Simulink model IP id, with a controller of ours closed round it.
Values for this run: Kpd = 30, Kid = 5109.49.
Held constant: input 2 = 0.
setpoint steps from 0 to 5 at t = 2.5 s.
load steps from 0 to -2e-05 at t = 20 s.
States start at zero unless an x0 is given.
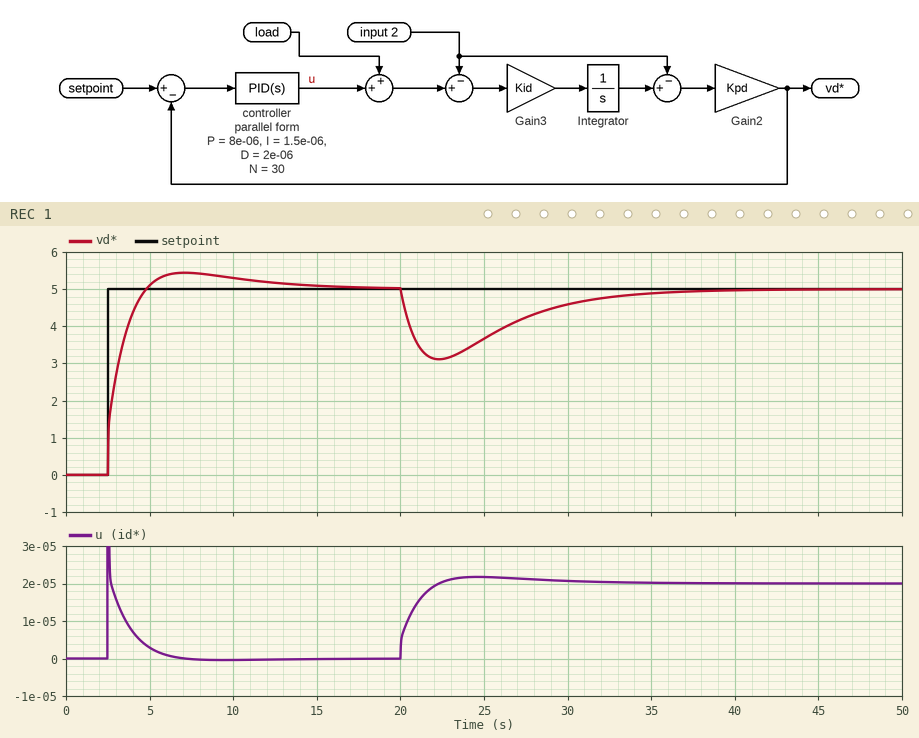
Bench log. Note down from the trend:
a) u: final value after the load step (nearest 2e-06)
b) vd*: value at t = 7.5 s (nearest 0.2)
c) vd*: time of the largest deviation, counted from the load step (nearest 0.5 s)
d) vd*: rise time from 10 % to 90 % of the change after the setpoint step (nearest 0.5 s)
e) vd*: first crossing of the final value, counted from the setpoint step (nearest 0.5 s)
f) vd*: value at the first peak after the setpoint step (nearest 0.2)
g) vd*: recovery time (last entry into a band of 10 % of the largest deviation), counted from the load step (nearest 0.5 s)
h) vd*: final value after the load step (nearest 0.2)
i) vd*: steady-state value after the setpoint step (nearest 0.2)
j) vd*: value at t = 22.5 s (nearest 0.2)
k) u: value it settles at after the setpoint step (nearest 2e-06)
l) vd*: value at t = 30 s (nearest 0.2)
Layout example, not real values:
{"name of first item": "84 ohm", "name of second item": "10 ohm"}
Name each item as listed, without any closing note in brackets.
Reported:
{"u: final value after the load step": "0.000020", "vd*: value at t = 7.5 s": "5.4", "vd*: time of the largest deviation, counted from the load step": "2.5 s", "vd*: rise time from 10 % to 90 % of the change after the setpoint step": "1.5 s", "vd*: first crossing of the final value, counted from the setpoint step": "2.5 s", "vd*: value at the first peak after the setpoint step": "5.4", "vd*: recovery time (last entry into a band of 10 % of the largest deviation), counted from the load step": "13.0 s", "vd*: final value after the load step": "5.0", "vd*: steady-state value after the setpoint step": "5.0", "vd*: value at t = 22.5 s": "3.2", "u: value it settles at after the setpoint step": "0.000000", "vd*: value at t = 30 s": "4.6"}
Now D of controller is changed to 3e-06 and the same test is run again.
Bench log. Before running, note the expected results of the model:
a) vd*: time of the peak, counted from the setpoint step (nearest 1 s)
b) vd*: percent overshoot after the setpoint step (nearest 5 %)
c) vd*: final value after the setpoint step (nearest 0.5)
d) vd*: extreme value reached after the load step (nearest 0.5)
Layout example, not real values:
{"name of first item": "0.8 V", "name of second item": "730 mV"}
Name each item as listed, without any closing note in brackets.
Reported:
{"vd*: time of the peak, counted from the setpoint step": "5 s", "vd*: percent overshoot after the setpoint step": "10 %", "vd*: final value after the setpoint step": "5.0", "vd*: extreme value reached after the load step": "3.0"}
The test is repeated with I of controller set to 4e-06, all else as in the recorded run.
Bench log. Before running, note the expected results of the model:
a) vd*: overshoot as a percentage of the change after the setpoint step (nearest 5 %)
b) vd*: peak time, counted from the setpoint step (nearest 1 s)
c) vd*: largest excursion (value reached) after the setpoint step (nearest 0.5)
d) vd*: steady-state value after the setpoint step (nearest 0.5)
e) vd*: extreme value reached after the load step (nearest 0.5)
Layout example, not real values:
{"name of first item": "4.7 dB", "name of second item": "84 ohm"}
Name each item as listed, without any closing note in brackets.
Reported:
{"vd*: overshoot as a percentage of the change after the setpoint step": "15 %", "vd*: peak time, counted from the setpoint step": "3 s", "vd*: largest excursion (value reached) after the setpoint step": "6.0", "vd*: steady-state value after the setpoint step": "5.0", "vd*: extreme value reached after the load step": "3.5"}
